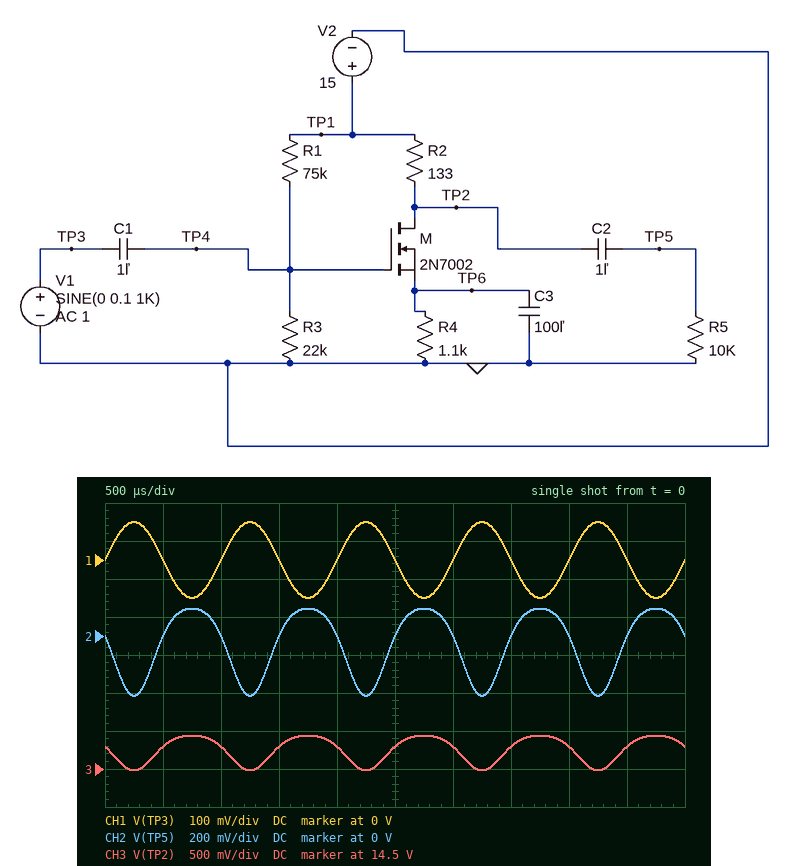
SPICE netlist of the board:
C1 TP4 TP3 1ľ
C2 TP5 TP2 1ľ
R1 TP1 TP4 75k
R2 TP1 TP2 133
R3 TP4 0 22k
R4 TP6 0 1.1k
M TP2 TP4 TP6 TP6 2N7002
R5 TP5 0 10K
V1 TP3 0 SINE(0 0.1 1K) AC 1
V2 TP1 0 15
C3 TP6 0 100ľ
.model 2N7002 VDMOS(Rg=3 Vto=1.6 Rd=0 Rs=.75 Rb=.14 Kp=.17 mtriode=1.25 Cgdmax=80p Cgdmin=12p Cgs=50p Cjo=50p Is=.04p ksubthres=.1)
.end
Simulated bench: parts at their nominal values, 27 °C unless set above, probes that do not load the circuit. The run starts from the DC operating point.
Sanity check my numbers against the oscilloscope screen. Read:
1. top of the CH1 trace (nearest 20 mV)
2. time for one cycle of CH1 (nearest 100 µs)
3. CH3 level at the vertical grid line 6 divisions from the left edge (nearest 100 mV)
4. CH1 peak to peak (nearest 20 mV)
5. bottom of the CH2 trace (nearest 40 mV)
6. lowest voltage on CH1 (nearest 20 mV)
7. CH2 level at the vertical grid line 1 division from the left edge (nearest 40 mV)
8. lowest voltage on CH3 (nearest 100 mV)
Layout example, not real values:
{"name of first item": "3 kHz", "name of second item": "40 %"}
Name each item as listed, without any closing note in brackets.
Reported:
{"top of the CH1 trace": "100 mV", "time for one cycle of CH1": "1.0 ms", "CH3 level at the vertical grid line 6 divisions from the left edge": "14.8 V", "CH1 peak to peak": "200 mV", "bottom of the CH2 trace": "-320 mV", "lowest voltage on CH1": "-100 mV", "CH2 level at the vertical grid line 1 division from the left edge": "0 V", "lowest voltage on CH3": "14.5 V"}
